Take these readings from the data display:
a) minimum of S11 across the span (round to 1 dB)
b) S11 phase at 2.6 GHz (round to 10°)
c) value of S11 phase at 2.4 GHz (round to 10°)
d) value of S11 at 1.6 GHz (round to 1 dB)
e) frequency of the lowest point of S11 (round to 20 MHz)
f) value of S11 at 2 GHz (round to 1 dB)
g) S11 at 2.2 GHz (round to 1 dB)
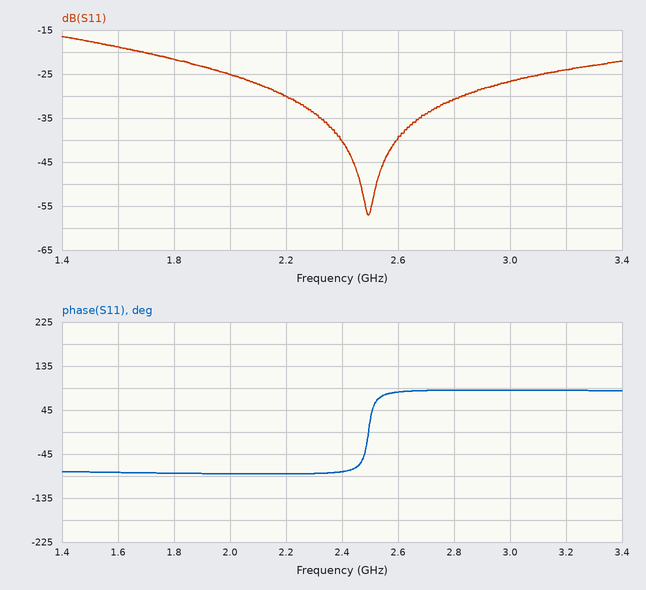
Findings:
-57 dB
80°
-80°
-19 dB
2.50 GHz
-25 dB
-30 dB
